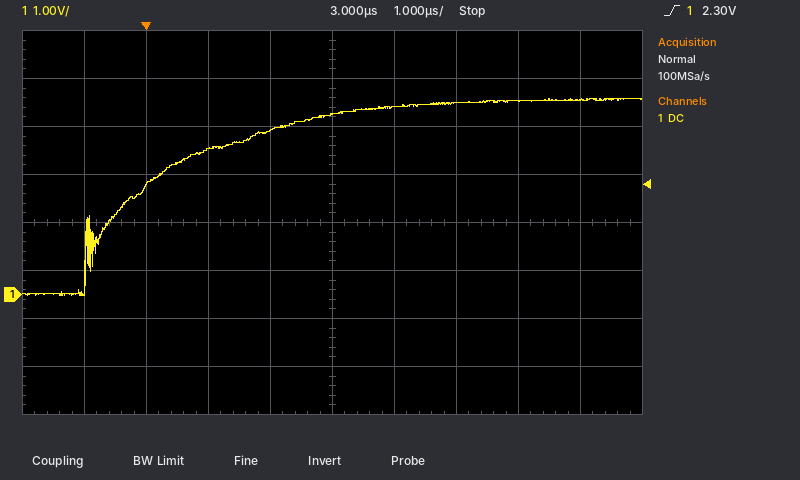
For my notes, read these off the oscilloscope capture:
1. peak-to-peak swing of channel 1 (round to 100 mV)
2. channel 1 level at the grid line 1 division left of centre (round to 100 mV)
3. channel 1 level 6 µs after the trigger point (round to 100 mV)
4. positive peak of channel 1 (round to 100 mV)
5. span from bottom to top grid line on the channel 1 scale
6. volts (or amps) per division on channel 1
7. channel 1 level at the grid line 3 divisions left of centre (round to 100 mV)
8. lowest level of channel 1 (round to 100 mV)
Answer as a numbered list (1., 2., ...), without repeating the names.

1. 4.1 V
2. 3.4 V
3. 4.0 V
4. 4.1 V
5. 8 V
6. 1 V
7. 2.3 V
8. 0.0 V
